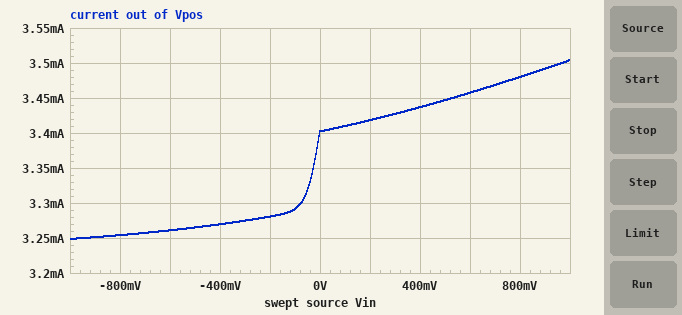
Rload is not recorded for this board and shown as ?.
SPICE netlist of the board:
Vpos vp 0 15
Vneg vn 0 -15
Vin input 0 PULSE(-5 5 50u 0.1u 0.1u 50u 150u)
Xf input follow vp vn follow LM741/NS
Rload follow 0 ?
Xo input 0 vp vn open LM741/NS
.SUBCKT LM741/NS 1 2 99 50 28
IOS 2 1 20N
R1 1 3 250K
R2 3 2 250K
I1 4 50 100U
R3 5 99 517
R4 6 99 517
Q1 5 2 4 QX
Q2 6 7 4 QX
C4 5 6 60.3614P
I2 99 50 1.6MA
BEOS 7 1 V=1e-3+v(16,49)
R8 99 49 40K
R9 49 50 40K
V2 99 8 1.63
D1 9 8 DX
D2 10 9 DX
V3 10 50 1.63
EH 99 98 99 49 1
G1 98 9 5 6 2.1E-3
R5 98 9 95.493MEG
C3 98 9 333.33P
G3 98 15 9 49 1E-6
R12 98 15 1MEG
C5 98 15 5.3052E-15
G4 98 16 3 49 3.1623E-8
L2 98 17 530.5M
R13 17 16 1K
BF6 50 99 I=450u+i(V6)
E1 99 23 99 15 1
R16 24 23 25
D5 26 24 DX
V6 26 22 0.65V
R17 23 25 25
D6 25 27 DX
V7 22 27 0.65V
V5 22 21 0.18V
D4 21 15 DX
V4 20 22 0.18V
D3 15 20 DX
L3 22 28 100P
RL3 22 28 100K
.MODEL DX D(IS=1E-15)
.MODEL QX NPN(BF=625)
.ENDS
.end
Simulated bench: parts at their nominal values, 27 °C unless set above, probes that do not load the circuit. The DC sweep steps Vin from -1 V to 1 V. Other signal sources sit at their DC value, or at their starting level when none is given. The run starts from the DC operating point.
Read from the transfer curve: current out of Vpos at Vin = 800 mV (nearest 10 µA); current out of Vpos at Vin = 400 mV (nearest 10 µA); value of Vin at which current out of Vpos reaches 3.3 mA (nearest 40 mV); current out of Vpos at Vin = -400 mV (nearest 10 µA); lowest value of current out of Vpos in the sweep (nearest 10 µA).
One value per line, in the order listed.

3.48 mA
3.44 mA
-80 mV
3.27 mA
3.25 mA
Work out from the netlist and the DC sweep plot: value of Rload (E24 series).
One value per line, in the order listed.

6.8 kΩ
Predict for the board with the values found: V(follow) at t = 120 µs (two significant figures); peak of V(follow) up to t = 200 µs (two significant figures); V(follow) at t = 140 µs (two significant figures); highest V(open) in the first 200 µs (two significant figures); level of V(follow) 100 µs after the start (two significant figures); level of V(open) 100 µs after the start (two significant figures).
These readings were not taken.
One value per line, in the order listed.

-1.3 V
5.0 V
-5.0 V
2.3 V
5.0 V
2.2 V
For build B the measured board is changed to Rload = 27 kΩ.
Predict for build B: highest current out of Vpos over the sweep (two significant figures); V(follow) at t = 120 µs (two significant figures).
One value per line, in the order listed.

3.4 mA
-1.4 V
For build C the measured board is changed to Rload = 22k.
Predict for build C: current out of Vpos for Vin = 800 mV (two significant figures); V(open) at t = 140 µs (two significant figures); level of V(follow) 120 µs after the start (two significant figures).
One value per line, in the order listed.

3.4 mA
-11 V
-1.4 V
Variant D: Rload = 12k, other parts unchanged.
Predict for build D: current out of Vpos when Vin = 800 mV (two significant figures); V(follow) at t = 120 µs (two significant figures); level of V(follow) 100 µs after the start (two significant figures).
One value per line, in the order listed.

3.4 mA
-1.4 V
5.0 V
